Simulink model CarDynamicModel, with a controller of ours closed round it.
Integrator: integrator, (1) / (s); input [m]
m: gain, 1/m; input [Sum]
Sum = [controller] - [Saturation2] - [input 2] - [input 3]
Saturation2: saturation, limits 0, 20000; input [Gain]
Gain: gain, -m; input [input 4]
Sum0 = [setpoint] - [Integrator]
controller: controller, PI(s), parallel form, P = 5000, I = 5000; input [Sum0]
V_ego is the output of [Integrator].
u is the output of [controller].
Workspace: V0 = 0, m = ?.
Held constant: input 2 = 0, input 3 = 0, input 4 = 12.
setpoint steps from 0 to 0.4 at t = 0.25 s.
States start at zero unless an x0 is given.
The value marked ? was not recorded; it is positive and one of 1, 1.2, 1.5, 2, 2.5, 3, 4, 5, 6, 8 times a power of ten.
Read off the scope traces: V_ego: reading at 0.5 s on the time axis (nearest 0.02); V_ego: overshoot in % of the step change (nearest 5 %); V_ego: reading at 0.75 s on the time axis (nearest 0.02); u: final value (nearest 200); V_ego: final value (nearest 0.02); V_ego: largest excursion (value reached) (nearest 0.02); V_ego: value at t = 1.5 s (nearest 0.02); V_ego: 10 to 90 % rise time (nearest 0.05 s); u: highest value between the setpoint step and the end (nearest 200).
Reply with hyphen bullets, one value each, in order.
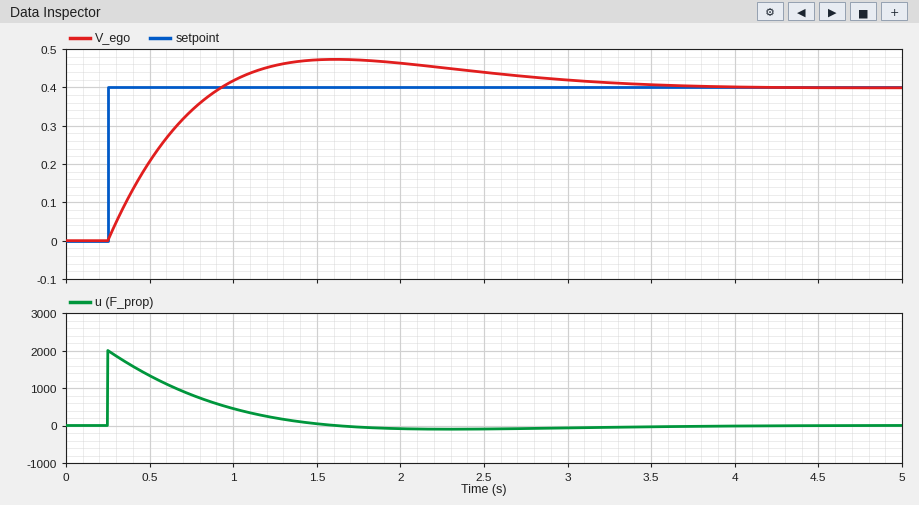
- 0.20
- 20 %
- 0.34
- 0
- 0.40
- 0.48
- 0.48
- 0.50 s
- 2000
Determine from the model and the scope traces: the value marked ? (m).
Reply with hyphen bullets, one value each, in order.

- 2000
